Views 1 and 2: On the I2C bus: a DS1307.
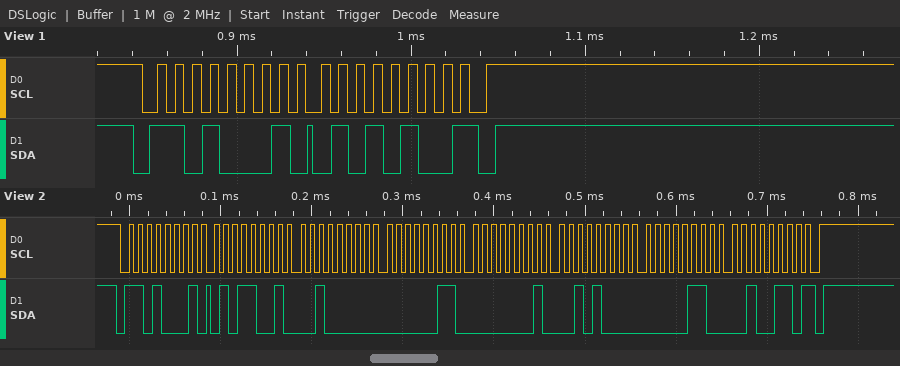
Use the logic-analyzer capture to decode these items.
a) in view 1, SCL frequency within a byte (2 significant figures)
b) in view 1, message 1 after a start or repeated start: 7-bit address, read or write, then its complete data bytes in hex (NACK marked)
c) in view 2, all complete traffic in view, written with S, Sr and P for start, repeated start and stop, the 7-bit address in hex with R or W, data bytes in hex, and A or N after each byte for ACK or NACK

100 kHz
0x68 read: 54 NACK
S 68R A 59 A 20 A 03 A 01 A 28 A 06 A 26 N P
